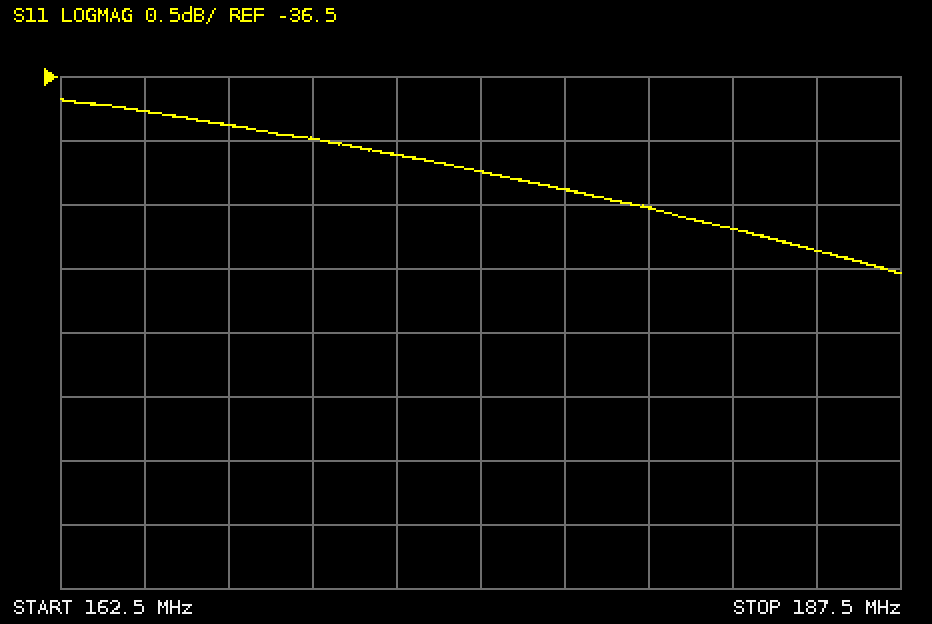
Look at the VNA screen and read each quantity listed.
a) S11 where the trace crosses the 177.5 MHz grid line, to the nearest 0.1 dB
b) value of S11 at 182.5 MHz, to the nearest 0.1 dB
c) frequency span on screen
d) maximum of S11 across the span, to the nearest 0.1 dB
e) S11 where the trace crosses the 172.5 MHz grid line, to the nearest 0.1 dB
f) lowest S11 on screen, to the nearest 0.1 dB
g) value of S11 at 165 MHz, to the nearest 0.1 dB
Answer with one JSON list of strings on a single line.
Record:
["-37.4 dB", "-37.7 dB", "25 MHz", "-36.7 dB", "-37.1 dB", "-38.0 dB", "-36.8 dB"]
